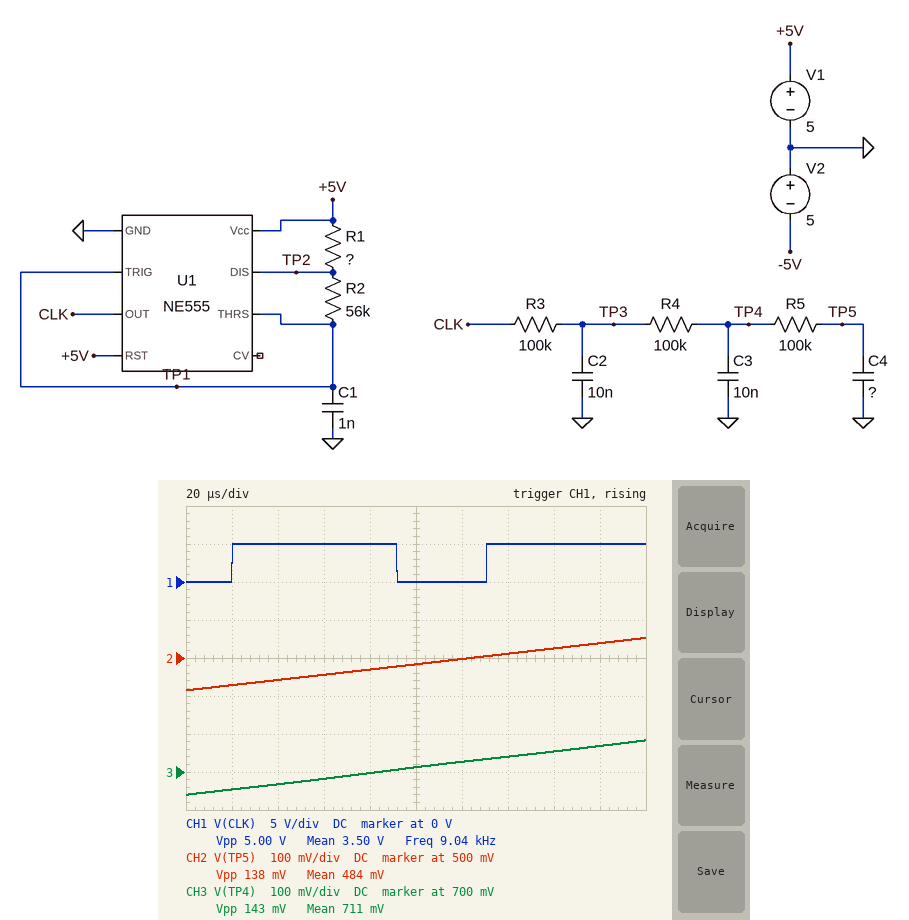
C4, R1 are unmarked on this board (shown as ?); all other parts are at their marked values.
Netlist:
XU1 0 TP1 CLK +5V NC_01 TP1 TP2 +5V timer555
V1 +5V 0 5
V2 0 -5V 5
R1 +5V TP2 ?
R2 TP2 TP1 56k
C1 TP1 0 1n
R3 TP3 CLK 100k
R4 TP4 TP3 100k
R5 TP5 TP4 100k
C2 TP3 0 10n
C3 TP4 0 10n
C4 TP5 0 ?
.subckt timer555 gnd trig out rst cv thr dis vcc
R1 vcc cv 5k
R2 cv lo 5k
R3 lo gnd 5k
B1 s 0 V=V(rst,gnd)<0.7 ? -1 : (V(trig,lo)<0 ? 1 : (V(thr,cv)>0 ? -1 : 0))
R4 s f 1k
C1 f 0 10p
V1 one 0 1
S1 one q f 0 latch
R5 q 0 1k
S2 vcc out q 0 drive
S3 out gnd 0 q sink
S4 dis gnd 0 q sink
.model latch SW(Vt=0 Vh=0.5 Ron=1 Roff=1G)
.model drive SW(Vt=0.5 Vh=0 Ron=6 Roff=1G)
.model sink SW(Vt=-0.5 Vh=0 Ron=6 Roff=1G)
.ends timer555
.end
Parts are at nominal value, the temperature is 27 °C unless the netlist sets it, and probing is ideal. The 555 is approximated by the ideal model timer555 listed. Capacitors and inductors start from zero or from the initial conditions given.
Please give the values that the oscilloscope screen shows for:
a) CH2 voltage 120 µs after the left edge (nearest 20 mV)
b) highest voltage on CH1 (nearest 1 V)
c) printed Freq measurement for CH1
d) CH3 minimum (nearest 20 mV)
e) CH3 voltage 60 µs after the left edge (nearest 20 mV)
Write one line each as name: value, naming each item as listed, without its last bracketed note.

CH2 voltage 120 µs after the left edge: 500 mV
highest voltage on CH1: 5 V
printed Freq measurement for CH1: 9.04 kHz
CH3 minimum: 640 mV
CH3 voltage 60 µs after the left edge: 680 mV
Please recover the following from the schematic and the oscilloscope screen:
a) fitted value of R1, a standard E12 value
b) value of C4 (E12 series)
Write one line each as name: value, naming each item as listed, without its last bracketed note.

fitted value of R1, a standard E12 value: 47 kΩ
value of C4: 3.3 nF
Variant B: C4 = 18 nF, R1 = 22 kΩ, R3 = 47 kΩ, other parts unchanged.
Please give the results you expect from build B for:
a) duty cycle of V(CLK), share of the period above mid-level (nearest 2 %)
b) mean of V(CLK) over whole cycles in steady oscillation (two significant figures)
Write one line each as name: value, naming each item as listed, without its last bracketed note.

duty cycle of V(CLK), share of the period above mid-level: 58 %
mean of V(CLK) over whole cycles in steady oscillation: 2.9 V
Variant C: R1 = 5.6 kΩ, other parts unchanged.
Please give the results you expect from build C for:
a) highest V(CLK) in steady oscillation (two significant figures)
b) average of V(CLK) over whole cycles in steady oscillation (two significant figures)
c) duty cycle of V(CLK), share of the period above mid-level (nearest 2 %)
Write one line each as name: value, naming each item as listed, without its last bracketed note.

highest V(CLK) in steady oscillation: 5.0 V
average of V(CLK) over whole cycles in steady oscillation: 2.6 V
duty cycle of V(CLK), share of the period above mid-level: 52 %
